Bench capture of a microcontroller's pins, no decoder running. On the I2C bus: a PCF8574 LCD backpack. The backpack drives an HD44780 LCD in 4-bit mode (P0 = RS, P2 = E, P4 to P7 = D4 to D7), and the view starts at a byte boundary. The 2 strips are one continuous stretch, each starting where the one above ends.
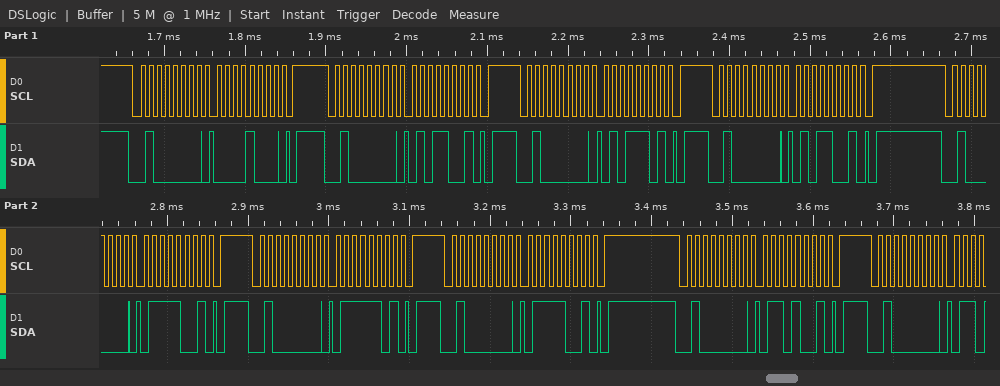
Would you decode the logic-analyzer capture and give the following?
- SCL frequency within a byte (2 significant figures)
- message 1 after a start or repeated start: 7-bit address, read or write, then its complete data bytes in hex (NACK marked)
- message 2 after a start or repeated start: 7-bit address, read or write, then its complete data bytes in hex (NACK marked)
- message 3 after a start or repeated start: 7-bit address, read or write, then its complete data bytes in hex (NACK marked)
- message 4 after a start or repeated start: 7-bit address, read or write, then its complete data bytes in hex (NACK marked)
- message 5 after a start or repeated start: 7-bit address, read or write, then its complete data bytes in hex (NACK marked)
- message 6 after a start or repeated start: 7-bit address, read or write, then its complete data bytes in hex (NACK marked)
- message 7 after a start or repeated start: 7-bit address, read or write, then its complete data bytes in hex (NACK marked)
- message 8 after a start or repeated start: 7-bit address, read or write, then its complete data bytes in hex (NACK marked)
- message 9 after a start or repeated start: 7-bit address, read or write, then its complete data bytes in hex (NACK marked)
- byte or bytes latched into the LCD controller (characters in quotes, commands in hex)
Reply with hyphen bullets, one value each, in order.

- 100 kHz
- 0x20 write: 08
- 0x20 write: 59
- 0x20 write: 5D
- 0x20 write: 59
- 0x20 write: 79
- 0x20 write: 7D
- 0x20 write: 79
- 0x20 write: 69
- 0x20 write
- 'W'
